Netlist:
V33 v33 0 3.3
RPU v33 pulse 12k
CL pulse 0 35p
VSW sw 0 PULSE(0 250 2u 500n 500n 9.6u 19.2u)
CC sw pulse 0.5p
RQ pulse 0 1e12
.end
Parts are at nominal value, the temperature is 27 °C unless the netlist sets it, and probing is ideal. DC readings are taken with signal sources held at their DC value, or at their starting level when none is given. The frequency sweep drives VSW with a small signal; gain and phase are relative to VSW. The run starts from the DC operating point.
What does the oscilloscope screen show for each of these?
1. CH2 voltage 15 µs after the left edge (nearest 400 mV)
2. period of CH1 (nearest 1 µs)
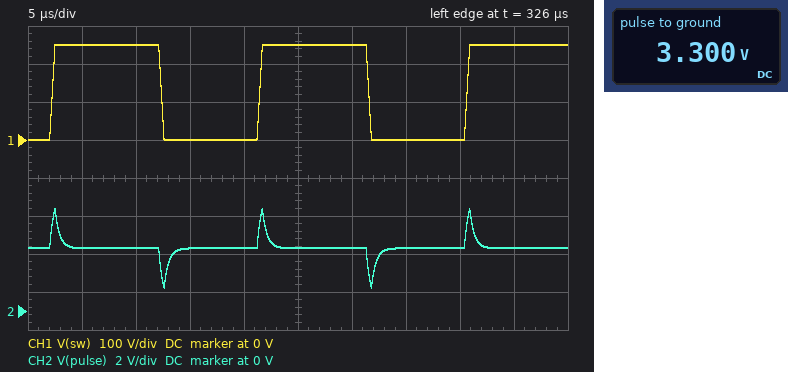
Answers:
3.2 V
19 µs
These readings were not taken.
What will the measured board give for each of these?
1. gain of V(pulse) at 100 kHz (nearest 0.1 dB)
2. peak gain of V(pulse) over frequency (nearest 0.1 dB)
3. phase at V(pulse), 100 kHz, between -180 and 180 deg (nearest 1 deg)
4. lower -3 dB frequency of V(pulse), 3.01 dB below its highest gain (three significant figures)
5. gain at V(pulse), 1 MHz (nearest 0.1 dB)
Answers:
-48.8 dB
-37.0 dB
75 deg
374 kHz
-37.6 dB
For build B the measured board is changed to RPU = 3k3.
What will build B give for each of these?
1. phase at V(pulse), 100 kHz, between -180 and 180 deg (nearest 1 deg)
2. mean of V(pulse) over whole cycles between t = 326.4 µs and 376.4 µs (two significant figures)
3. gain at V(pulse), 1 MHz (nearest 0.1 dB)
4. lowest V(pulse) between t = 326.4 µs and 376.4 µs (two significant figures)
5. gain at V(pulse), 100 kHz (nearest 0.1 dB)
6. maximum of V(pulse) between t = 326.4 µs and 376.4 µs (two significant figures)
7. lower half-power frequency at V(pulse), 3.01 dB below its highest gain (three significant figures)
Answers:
86 deg
3.3 V
-41.6 dB
2.5 V
-59.7 dB
4.1 V
1.36 MHz
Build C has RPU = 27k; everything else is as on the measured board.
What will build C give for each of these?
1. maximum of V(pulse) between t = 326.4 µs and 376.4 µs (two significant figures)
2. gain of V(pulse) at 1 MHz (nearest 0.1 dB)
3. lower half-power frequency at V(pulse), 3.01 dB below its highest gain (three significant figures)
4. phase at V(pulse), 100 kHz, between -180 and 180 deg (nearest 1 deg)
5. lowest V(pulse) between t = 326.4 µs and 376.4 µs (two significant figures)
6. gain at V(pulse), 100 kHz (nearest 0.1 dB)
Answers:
6.0 V
-37.1 dB
166 kHz
59 deg
560 mV
-42.8 dB
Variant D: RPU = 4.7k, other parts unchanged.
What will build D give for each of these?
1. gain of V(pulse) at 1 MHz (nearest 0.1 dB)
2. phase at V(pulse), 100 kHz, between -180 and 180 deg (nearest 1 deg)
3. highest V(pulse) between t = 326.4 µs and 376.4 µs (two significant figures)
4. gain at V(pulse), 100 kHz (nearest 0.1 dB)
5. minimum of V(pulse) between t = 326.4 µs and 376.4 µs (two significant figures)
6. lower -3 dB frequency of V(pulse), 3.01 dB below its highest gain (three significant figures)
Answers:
-39.8 dB
84 deg
4.4 V
-56.7 dB
2.2 V
954 kHz
